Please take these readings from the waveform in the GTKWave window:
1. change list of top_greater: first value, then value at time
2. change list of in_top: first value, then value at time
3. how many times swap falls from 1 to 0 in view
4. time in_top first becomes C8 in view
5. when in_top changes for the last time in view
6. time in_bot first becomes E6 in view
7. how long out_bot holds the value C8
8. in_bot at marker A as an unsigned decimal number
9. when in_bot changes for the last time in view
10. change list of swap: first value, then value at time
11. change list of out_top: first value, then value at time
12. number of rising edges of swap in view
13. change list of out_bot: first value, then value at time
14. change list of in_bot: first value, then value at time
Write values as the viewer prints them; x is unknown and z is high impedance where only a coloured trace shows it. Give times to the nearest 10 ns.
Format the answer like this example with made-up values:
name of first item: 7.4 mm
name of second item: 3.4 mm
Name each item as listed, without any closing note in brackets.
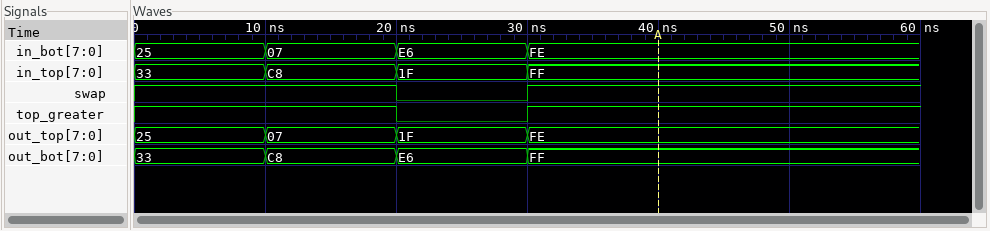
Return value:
change list of top_greater: first value, then value at time: 1, 0 at 20 ns, 1 at 30 ns
change list of in_top: first value, then value at time: 33, C8 at 10 ns, 1F at 20 ns, FF at 30 ns
how many times swap falls from 1 to 0 in view: 1
time in_top first becomes C8 in view: 10 ns
when in_top changes for the last time in view: 30 ns
time in_bot first becomes E6 in view: 20 ns
how long out_bot holds the value C8: 10 ns
in_bot at marker A as an unsigned decimal number: 254
when in_bot changes for the last time in view: 30 ns
change list of swap: first value, then value at time: 1, 0 at 20 ns, 1 at 30 ns
change list of out_top: first value, then value at time: 25, 07 at 10 ns, 1F at 20 ns, FE at 30 ns
number of rising edges of swap in view: 1
change list of out_bot: first value, then value at time: 33, C8 at 10 ns, E6 at 20 ns, FF at 30 ns
change list of in_bot: first value, then value at time: 25, 07 at 10 ns, E6 at 20 ns, FE at 30 ns
